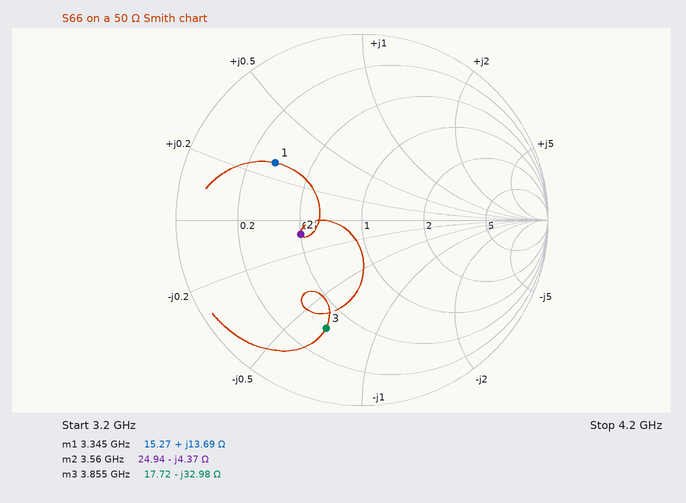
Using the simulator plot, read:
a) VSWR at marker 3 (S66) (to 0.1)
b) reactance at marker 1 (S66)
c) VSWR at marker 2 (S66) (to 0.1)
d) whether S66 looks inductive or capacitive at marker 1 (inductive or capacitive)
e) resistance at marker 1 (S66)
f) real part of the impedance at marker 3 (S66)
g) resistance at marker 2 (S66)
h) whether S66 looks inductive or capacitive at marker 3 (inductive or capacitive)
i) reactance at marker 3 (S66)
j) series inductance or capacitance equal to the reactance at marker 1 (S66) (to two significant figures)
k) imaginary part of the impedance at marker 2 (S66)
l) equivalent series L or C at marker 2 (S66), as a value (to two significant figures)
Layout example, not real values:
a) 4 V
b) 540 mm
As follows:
a) 4.2
b) +13.69 Ω
c) 2.0
d) inductive
e) 15.27 Ω
f) 17.72 Ω
g) 24.94 Ω
h) capacitive
i) -32.98 Ω
j) 650 pH
k) -4.37 Ω
l) 10 pF
